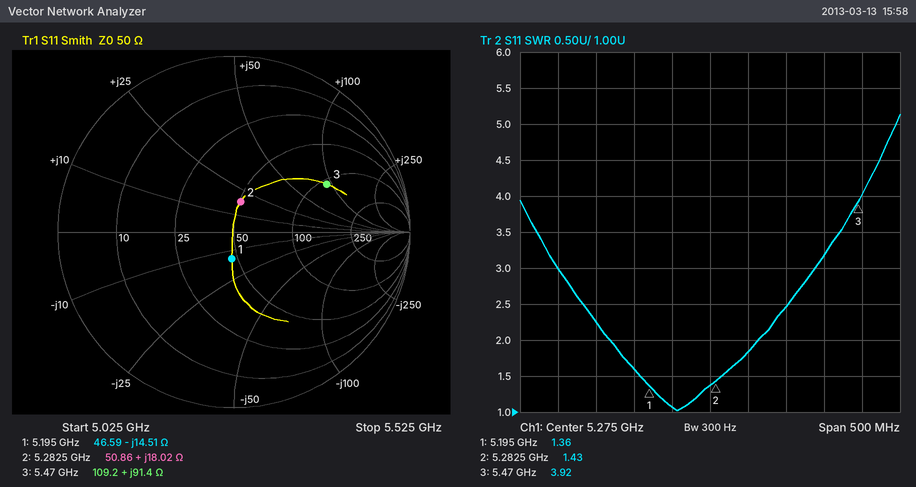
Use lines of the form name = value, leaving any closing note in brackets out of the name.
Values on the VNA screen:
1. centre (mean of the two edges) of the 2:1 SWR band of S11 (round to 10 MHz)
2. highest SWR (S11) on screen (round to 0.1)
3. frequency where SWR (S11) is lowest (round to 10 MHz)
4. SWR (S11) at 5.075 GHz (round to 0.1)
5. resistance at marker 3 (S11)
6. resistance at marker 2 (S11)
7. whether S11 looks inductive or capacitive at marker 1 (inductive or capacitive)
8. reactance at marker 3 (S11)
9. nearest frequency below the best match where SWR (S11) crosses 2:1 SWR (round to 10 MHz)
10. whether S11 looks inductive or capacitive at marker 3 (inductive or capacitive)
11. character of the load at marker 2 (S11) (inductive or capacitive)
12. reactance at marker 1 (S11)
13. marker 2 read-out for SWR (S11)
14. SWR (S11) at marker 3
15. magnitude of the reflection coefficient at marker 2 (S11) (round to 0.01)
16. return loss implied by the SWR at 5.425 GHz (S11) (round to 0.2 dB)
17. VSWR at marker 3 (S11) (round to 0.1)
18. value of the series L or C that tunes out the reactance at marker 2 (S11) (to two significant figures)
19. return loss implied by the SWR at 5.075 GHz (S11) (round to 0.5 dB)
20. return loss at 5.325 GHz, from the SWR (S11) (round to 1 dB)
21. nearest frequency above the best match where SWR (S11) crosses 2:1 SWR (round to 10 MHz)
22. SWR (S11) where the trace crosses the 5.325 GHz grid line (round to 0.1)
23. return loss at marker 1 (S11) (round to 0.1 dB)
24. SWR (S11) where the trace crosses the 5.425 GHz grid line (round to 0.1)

centre (mean of the two edges) of the 2:1 SWR band of S11 = 5.24 GHz
highest SWR (S11) on screen = 5.1
frequency where SWR (S11) is lowest = 5.23 GHz
SWR (S11) at 5.075 GHz = 3.0
resistance at marker 3 = 109.2 Ω
resistance at marker 2 = 50.86 Ω
whether S11 looks inductive or capacitive at marker 1 = capacitive
reactance at marker 3 = +91.4 Ω
nearest frequency below the best match where SWR (S11) crosses 2:1 SWR = 5.14 GHz
whether S11 looks inductive or capacitive at marker 3 = inductive
character of the load at marker 2 (S11) = inductive
reactance at marker 1 = -14.51 Ω
marker 2 read-out for SWR = 1.43
SWR (S11) at marker 3 = 3.92
magnitude of the reflection coefficient at marker 2 (S11) = 0.18
return loss implied by the SWR at 5.425 GHz (S11) = 5.6 dB
VSWR at marker 3 (S11) = 3.9
value of the series L or C that tunes out the reactance at marker 2 (S11) = 1.7 pF
return loss implied by the SWR at 5.075 GHz (S11) = 6.0 dB
return loss at 5.325 GHz, from the SWR (S11) = 11 dB
nearest frequency above the best match where SWR (S11) crosses 2:1 SWR = 5.34 GHz
SWR (S11) where the trace crosses the 5.325 GHz grid line = 1.8
return loss at marker 1 (S11) = 16.3 dB
SWR (S11) where the trace crosses the 5.425 GHz grid line = 3.2
